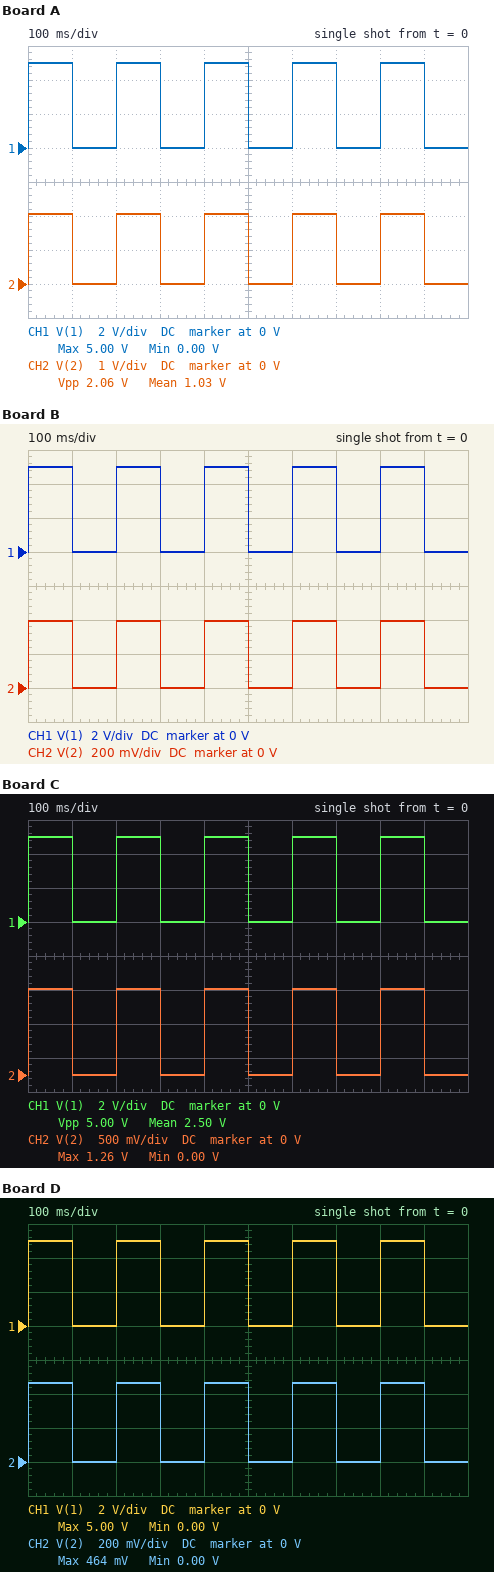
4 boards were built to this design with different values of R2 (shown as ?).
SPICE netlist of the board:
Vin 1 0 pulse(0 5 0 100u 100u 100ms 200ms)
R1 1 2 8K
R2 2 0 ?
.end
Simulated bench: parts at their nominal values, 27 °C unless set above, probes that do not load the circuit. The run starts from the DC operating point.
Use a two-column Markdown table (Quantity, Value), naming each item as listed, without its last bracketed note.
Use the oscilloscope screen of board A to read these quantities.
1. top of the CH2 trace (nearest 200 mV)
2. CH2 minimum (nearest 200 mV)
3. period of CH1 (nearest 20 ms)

| Quantity | Value |
|---|---|
| top of the CH2 trace | 2.0 V |
| CH2 minimum | 0 V |
| period of CH1 | 200 ms |
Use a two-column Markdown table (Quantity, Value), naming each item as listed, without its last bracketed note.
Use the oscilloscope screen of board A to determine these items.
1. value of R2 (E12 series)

| Quantity | Value |
|---|---|
| value of R2 | 5.6 kΩ |
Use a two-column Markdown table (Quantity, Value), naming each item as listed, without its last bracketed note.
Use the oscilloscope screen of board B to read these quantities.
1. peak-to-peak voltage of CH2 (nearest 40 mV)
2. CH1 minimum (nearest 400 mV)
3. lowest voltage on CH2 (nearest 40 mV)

| Quantity | Value |
|---|---|
| peak-to-peak voltage of CH2 | 400 mV |
| CH1 minimum | 0 V |
| lowest voltage on CH2 | 0 V |
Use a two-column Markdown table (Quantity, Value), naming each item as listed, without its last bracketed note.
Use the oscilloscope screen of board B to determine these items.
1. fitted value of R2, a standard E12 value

| Quantity | Value |
|---|---|
| fitted value of R2, a standard E12 value | 680 Ω |
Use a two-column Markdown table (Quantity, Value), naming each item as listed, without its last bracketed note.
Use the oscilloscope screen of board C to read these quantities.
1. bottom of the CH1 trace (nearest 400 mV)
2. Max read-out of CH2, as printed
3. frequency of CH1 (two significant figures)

| Quantity | Value |
|---|---|
| bottom of the CH1 trace | 0 V |
| Max read-out of CH2, as printed | 1.26 V |
| frequency of CH1 | 5.0 Hz |
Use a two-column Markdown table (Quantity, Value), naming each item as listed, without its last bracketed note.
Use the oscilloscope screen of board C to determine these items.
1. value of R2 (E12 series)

| Quantity | Value |
|---|---|
| value of R2 | 2.7 kΩ |
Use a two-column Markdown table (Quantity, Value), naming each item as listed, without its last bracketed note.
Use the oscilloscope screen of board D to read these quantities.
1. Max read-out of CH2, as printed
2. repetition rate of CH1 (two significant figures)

| Quantity | Value |
|---|---|
| Max read-out of CH2, as printed | 464 mV |
| repetition rate of CH1 | 5.0 Hz |
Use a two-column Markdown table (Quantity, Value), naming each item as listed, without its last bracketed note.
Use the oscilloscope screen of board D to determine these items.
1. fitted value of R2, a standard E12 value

| Quantity | Value |
|---|---|
| fitted value of R2, a standard E12 value | 820 Ω |
